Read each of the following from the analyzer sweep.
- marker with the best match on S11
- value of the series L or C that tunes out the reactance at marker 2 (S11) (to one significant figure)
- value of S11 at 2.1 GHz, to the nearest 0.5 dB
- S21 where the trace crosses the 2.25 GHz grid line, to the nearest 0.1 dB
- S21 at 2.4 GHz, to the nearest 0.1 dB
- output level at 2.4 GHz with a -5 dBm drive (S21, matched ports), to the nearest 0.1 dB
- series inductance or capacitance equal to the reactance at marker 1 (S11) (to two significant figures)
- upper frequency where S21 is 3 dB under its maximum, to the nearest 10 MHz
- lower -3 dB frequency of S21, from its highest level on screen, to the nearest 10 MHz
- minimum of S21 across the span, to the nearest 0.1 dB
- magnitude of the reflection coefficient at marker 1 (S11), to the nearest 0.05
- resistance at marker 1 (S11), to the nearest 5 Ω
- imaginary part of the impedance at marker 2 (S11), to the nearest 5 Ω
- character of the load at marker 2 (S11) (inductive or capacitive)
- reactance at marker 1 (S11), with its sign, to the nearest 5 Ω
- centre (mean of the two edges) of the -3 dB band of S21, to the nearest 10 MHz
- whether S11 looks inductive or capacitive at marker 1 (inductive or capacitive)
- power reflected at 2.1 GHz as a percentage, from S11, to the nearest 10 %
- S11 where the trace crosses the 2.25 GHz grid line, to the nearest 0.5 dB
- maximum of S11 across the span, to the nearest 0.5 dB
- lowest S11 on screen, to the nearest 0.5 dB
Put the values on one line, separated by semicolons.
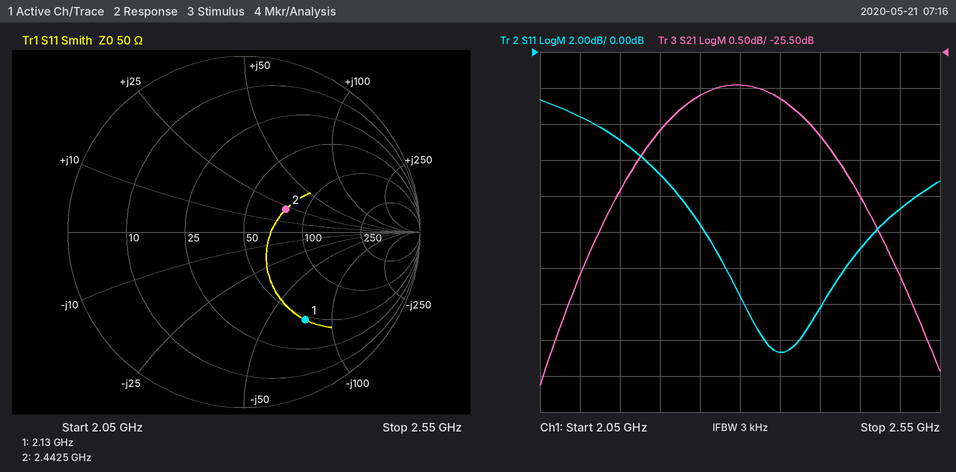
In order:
marker 2; 3 pF; -3.5 dB; -26.1 dB; -26.7 dB; -31.7 dBm; 1.0 pF; 2.51 GHz; 2.09 GHz; -30.1 dB; 0.60; 45 Ω; +20 Ω; inductive; -75 Ω; 2.30 GHz; capacitive; 40 %; -9.5 dB; -2.5 dB; -16.5 dB
